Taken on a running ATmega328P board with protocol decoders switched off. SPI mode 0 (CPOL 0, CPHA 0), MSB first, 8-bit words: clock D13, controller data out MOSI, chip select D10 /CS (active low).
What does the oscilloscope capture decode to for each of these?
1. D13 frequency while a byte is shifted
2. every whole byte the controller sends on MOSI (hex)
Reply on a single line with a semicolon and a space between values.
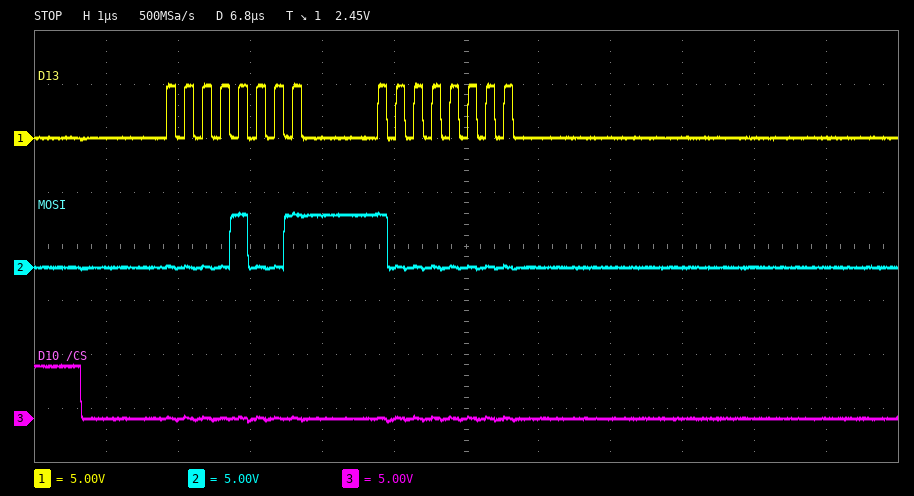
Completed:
4 MHz; 09 80
